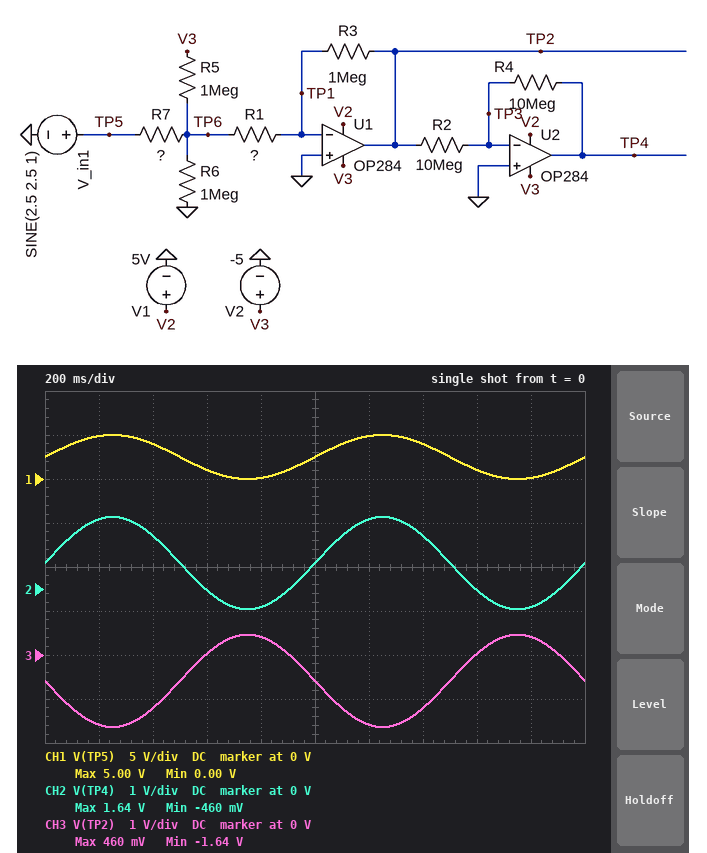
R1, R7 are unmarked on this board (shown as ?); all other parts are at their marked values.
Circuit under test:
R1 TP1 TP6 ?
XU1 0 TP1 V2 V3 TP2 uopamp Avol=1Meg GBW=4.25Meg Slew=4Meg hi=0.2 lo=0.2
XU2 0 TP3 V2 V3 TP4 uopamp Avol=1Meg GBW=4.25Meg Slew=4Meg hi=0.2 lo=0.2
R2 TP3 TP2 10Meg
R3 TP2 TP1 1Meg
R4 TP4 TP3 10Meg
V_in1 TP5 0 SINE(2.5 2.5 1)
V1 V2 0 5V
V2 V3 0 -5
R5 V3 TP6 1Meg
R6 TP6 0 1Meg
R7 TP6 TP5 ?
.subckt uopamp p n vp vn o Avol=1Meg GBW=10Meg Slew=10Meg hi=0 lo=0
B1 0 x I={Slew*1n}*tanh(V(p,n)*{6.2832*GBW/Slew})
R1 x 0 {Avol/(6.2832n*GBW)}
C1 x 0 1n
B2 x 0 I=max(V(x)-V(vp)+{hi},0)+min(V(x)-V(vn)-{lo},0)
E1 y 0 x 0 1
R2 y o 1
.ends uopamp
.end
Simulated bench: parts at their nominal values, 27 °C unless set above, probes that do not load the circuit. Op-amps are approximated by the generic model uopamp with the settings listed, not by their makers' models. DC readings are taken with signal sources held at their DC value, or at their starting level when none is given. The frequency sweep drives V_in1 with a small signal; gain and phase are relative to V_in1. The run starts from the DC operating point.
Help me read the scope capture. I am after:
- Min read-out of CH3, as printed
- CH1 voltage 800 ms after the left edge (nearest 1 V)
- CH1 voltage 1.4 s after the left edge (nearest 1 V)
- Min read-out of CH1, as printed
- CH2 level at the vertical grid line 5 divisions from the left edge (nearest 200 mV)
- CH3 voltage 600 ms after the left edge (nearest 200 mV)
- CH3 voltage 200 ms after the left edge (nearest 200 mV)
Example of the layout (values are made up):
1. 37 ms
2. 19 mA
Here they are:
1. -1.64 V
2. 0 V
3. 4 V
4. 0.00 V
5. 600 mV
6. 0 V
7. -1.6 V
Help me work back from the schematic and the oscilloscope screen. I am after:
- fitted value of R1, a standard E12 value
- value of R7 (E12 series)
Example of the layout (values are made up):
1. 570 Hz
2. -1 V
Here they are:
1. 1.5 MΩ
2. 220 kΩ
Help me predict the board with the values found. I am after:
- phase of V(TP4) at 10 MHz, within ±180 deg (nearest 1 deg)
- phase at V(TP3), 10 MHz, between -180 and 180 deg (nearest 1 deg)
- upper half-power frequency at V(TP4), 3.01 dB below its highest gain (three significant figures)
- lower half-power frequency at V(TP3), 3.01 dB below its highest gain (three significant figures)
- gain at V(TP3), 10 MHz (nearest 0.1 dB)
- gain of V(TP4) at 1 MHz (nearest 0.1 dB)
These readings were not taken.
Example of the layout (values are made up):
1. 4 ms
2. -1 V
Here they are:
1. -153 deg
2. 117 deg
3. 1.51 MHz
4. 978 kHz
5. -25.6 dB
6. -9.0 dB
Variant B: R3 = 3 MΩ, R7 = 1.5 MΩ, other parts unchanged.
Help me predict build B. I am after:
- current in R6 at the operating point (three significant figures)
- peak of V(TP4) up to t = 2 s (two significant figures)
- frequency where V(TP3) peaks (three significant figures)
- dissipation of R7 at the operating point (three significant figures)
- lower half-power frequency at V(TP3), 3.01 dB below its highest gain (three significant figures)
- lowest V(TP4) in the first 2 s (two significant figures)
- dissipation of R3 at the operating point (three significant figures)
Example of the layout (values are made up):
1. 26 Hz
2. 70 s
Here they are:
1. 1.00 µA
2. -1.0 V
3. 1.86 MHz
4. 8.17 µW
5. 767 kHz
6. -3.0 V
7. 1.33 µW
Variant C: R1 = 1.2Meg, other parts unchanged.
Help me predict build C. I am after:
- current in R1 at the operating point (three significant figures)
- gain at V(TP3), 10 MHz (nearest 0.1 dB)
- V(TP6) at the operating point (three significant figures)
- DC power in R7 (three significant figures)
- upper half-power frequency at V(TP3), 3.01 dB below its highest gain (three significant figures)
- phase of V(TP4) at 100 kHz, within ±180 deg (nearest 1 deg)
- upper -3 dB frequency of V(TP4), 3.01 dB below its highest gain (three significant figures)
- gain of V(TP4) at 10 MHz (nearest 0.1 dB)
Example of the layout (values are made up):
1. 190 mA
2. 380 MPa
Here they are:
1. 719 nA
2. -24.5 dB
3. 862 mV
4. 12.2 µW
5. 5.51 MHz
6. -5 deg
7. 1.46 MHz
8. -31.9 dB
